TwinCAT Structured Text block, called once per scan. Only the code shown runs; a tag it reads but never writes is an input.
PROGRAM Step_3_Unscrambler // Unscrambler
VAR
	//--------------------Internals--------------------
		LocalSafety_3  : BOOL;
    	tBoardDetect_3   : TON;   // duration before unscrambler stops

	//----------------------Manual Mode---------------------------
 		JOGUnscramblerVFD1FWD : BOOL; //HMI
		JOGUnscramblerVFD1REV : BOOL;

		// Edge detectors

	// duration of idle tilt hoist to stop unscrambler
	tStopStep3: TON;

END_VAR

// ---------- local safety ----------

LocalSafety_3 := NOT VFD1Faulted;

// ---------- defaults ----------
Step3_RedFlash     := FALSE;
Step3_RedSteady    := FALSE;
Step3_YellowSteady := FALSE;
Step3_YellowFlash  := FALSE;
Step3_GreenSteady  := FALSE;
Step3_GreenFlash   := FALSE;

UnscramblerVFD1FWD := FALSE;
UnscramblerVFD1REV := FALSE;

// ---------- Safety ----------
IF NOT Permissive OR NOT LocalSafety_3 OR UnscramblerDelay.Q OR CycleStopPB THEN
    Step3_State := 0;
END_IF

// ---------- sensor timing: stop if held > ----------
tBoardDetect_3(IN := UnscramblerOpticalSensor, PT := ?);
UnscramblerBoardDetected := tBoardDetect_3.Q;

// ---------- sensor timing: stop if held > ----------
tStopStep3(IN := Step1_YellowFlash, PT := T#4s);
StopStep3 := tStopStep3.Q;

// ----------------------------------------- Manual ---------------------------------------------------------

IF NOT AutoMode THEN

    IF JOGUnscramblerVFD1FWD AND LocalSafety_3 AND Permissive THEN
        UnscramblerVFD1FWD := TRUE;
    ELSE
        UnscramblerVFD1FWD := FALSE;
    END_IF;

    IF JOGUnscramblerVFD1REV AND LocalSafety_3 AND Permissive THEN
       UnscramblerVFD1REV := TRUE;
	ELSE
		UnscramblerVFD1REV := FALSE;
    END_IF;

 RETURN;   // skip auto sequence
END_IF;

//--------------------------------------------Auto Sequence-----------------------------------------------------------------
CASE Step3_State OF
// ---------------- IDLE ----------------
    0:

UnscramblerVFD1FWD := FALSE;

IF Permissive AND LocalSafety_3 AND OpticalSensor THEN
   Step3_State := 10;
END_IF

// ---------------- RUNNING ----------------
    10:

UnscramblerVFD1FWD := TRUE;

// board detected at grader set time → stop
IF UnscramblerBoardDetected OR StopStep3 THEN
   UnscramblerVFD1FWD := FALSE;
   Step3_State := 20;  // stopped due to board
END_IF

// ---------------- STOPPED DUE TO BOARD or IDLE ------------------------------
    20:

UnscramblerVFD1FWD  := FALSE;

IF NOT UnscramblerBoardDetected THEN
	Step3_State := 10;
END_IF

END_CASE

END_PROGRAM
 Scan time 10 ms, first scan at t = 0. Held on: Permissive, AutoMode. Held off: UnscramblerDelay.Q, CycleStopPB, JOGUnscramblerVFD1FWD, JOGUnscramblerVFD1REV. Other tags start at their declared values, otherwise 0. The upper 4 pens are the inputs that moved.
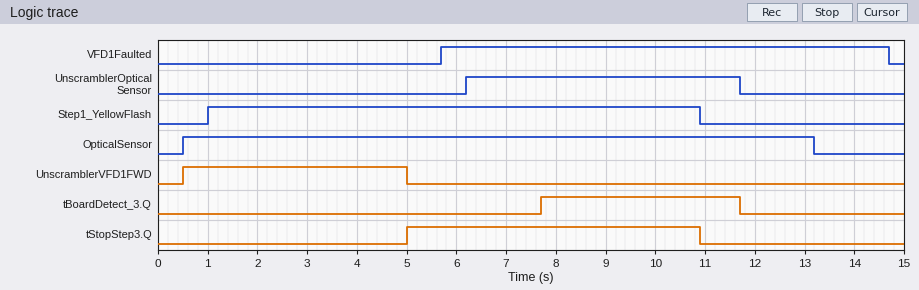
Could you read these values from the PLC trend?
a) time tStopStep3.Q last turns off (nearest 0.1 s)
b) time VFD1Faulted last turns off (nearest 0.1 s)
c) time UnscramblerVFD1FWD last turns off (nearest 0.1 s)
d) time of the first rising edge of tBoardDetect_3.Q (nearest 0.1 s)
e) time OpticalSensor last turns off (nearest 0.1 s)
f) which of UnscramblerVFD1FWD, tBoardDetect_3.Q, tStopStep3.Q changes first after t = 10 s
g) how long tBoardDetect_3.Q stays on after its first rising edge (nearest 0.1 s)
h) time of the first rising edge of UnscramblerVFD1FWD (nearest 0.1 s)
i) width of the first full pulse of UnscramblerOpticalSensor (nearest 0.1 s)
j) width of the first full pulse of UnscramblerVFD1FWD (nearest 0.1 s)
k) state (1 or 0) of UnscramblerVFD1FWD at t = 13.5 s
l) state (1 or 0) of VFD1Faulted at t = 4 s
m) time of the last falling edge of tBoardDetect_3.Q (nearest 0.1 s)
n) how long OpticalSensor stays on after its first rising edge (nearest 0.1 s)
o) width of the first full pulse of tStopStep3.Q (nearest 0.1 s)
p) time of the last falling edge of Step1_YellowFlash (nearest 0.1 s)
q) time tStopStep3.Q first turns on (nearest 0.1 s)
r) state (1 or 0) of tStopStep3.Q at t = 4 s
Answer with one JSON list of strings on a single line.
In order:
["10.9 s", "14.7 s", "5.0 s", "7.7 s", "13.2 s", "tStopStep3.Q", "4.0 s", "0.5 s", "5.5 s", "4.5 s", "0", "0", "11.7 s", "12.7 s", "5.9 s", "10.9 s", "5.0 s", "0"]
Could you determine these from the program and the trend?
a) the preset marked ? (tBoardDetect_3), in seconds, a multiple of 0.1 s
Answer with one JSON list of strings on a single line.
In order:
["1.5 s"]
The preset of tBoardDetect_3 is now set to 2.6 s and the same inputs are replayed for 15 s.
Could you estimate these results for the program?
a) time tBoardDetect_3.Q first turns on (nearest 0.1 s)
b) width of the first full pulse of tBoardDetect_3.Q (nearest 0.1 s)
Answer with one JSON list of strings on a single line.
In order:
["8.8 s", "2.9 s"]
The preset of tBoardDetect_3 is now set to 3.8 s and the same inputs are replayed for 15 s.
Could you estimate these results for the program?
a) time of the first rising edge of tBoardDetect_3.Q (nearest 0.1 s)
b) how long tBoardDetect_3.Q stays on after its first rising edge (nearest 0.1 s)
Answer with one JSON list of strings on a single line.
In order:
["10.0 s", "1.7 s"]
